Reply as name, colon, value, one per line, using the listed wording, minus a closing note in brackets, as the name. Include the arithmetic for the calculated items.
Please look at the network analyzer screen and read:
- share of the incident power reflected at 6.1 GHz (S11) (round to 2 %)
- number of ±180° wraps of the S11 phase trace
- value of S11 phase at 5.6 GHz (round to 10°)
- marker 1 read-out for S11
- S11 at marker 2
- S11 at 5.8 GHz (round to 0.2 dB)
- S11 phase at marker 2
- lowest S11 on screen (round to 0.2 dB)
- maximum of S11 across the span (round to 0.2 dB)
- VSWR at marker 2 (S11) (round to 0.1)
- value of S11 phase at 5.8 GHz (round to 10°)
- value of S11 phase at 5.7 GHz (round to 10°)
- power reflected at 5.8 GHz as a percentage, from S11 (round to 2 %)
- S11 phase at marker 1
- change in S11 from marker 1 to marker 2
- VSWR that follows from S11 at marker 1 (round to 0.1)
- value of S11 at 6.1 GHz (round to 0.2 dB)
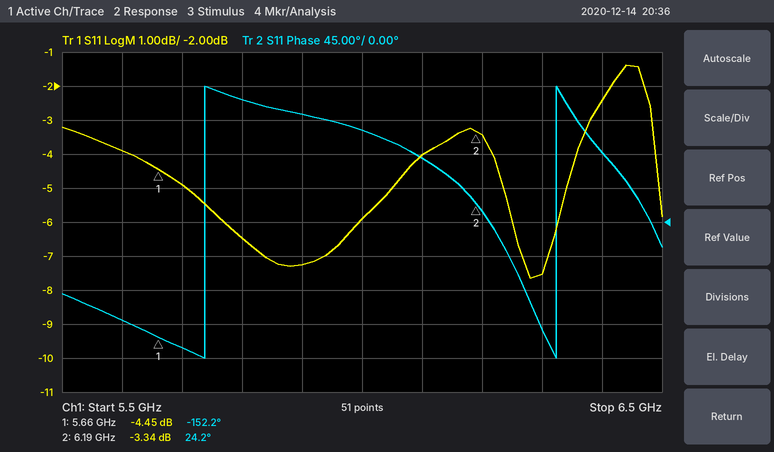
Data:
share of the incident power reflected at 6.1 GHz (S11): 10^(-4/10) ≈ 40 %
number of ±180° wraps of the S11 phase trace: 2
value of S11 phase at 5.6 GHz: -130°
marker 1 read-out for S11: -4.45 dB
S11 at marker 2: -3.34 dB
S11 at 5.8 GHz: -6.4 dB
S11 phase at marker 2: 24.2°
lowest S11 on screen: -7.6 dB
maximum of S11 across the span: -1.4 dB
VSWR at marker 2 (S11): (1 + 0.6808)/(1 − 0.6808) ≈ 5.3
value of S11 phase at 5.8 GHz: 160°
value of S11 phase at 5.7 GHz: -170°
power reflected at 5.8 GHz as a percentage, from S11: 10^(-6.4/10) ≈ 22.9 %, so 22 % to the nearest 2 %
S11 phase at marker 1: -152.2°
change in S11 from marker 1 to marker 2: -3.34 − (-4.45) = 1.11 dB
VSWR that follows from S11 at marker 1: (1 + 0.5991)/(1 − 0.5991) ≈ 4.0
value of S11 at 6.1 GHz: -4.0 dB
